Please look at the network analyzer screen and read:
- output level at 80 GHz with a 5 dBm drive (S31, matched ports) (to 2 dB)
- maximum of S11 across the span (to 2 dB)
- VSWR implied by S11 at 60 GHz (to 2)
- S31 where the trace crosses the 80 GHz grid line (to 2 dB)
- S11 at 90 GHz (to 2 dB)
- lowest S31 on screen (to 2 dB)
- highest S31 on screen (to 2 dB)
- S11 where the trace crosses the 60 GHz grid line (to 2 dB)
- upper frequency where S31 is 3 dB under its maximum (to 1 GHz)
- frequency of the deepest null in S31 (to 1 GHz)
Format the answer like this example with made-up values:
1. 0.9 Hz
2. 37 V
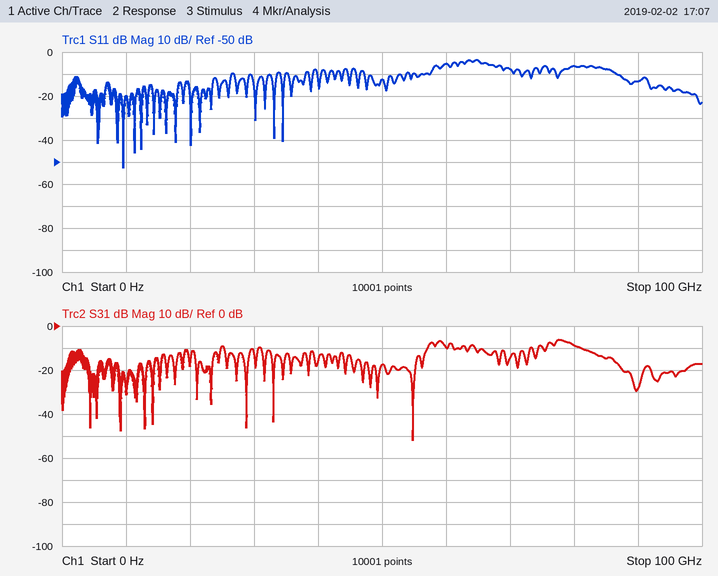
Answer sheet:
1. -4 dBm
2. -4 dB
3. 4
4. -8 dB
5. -14 dB
6. -52 dB
7. -6 dB
8. -6 dB
9. 80 GHz
10. 55 GHz
